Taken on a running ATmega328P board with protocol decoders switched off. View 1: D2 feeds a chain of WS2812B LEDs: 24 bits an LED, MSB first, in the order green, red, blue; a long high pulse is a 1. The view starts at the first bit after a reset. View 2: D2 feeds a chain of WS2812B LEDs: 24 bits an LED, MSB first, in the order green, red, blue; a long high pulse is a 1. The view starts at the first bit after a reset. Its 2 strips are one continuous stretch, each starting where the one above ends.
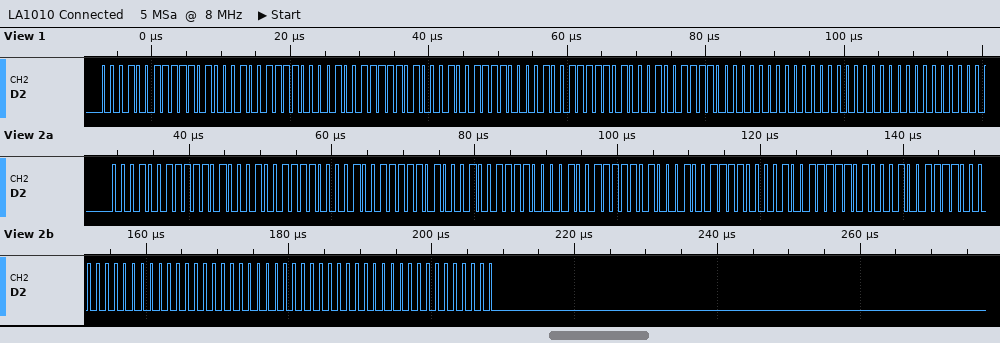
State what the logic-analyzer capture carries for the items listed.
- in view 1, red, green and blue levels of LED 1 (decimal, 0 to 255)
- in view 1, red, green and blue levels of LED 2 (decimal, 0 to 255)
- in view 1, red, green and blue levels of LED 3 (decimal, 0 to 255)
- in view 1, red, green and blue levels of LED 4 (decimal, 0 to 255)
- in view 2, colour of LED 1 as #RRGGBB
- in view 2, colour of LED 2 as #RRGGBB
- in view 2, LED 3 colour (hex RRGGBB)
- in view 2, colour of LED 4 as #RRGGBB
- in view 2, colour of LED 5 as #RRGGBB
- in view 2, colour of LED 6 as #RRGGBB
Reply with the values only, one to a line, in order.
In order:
232, 19, 158
232, 19, 158
232, 19, 158
0, 0, 0
#E8139E
#E8139E
#E8139E
#E8139E
#000000
#000000
